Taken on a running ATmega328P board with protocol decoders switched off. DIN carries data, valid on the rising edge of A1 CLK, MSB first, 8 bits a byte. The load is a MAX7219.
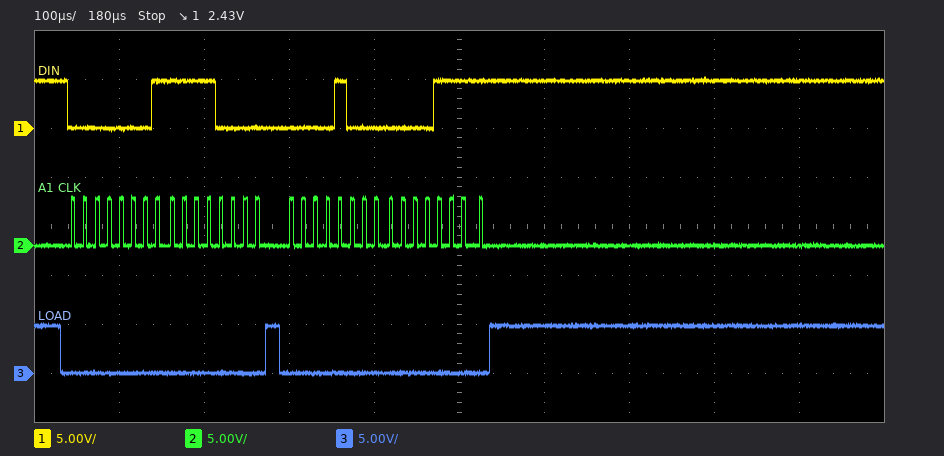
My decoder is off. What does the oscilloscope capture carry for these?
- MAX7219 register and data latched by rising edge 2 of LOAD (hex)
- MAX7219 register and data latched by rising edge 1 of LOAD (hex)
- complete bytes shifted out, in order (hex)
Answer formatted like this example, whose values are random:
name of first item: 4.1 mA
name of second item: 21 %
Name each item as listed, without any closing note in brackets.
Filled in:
MAX7219 register and data latched by rising edge 2 of LOAD: register 0x8, data 0x0F
MAX7219 register and data latched by rising edge 1 of LOAD: register 0x1, data 0xF0
complete bytes shifted out, in order: 01 F0 08 0F
